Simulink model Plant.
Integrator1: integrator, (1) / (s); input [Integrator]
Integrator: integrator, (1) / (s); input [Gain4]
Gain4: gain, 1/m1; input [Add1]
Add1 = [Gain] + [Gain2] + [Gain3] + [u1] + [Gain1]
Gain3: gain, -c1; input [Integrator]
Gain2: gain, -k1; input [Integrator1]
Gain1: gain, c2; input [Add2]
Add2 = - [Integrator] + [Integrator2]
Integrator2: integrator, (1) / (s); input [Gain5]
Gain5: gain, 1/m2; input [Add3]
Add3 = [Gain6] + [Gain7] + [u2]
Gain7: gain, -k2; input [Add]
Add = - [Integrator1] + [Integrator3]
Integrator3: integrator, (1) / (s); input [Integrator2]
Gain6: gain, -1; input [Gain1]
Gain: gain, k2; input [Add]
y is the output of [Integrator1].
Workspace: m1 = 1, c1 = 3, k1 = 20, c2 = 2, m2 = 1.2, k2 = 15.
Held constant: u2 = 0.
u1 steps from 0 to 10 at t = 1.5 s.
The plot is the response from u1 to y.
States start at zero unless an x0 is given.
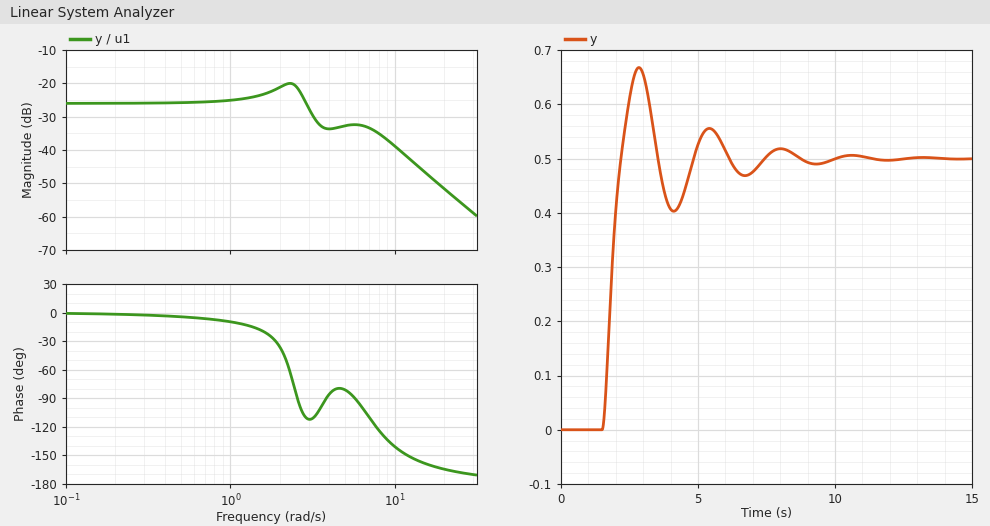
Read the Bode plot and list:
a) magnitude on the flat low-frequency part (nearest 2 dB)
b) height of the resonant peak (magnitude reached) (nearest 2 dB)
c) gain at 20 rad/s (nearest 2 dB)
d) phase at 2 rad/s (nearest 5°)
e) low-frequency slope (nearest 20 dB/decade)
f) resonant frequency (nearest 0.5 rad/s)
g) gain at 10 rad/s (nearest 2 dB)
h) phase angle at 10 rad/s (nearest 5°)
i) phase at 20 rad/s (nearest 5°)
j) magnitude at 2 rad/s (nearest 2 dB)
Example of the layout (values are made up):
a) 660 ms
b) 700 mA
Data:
a) -26 dB
b) -20 dB
c) -52 dB
d) -35°
e) 0 dB/decade
f) 2.5 rad/s
g) -38 dB
h) -140°
i) -165°
j) -22 dB
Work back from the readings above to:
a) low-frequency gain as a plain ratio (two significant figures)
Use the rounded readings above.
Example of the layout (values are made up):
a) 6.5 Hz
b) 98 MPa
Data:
a) 0.050
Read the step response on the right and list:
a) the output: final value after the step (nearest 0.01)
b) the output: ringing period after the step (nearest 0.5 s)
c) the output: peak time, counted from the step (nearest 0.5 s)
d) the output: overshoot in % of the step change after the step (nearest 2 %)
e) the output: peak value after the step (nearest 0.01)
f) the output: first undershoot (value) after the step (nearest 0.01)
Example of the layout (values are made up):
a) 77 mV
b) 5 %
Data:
a) 0.50
b) 2.5 s
c) 1.5 s
d) 34 %
e) 0.67
f) 0.40
